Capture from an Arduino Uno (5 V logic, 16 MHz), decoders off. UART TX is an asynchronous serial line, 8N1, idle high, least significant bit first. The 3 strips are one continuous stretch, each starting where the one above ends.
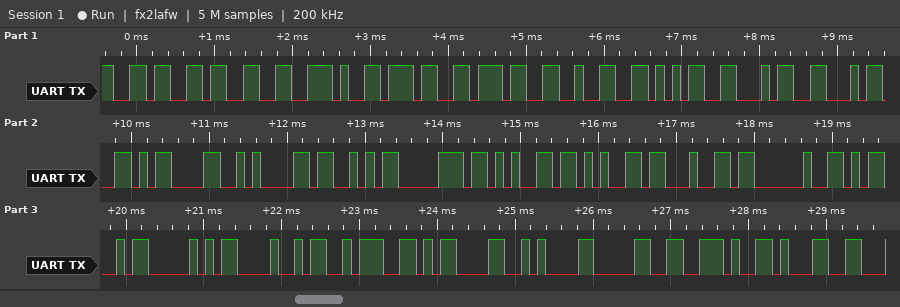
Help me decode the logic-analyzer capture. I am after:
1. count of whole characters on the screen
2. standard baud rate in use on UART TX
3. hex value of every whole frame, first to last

26
9600 baud
36 33 2E 37 37 32 35 34 34 0D 0A 53 70 65 65 64 20 4D 50 48 3A 0D 0A 30 2E 31
